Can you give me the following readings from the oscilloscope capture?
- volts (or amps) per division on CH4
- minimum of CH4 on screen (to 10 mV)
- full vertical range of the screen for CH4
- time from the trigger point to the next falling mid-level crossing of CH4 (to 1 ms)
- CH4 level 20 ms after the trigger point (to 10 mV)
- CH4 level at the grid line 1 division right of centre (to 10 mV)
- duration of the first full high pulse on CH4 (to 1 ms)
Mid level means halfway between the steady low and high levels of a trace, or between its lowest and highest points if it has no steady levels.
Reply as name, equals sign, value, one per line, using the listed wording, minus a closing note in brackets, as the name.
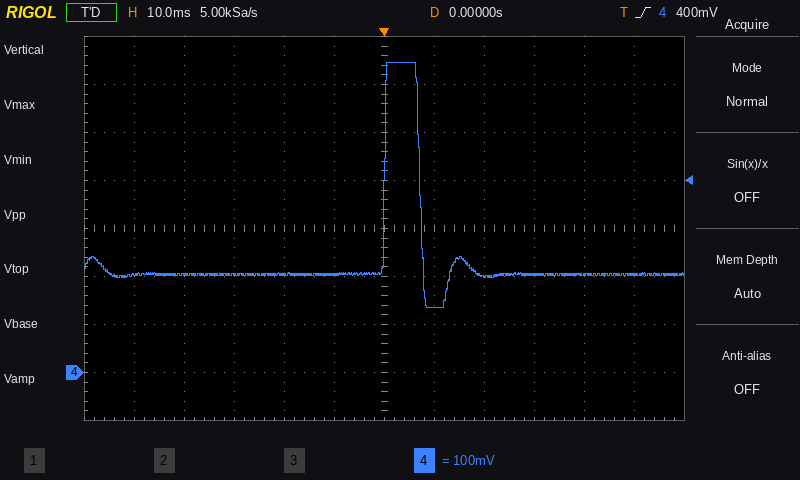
volts (or amps) per division on CH4 = 100 mV
minimum of CH4 on screen = 140 mV
full vertical range of the screen for CH4 = 800 mV
time from the trigger point to the next falling mid-level crossing of CH4 = 7 ms
CH4 level 20 ms after the trigger point = 200 mV
CH4 level at the grid line 1 division right of centre = 140 mV
duration of the first full high pulse on CH4 = 7 ms
